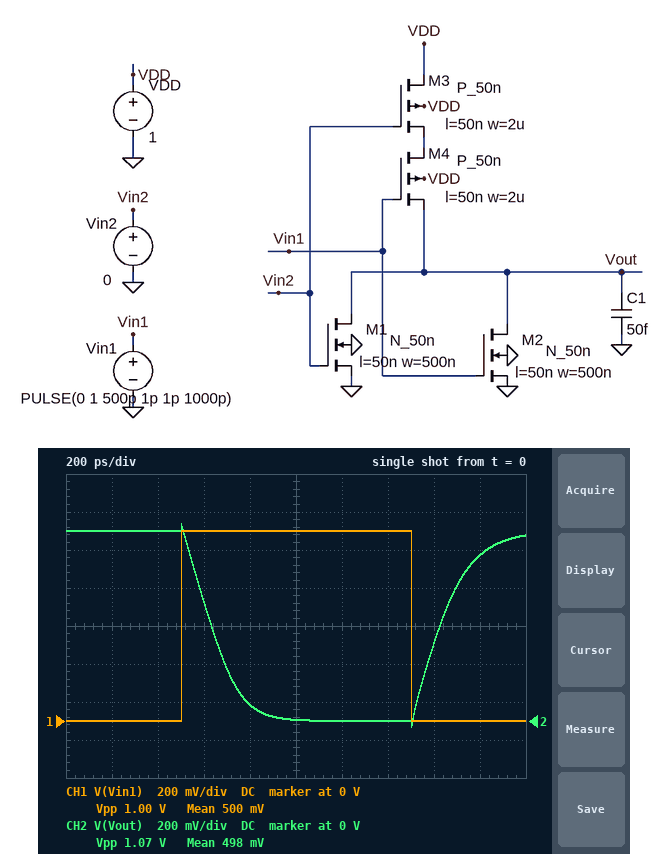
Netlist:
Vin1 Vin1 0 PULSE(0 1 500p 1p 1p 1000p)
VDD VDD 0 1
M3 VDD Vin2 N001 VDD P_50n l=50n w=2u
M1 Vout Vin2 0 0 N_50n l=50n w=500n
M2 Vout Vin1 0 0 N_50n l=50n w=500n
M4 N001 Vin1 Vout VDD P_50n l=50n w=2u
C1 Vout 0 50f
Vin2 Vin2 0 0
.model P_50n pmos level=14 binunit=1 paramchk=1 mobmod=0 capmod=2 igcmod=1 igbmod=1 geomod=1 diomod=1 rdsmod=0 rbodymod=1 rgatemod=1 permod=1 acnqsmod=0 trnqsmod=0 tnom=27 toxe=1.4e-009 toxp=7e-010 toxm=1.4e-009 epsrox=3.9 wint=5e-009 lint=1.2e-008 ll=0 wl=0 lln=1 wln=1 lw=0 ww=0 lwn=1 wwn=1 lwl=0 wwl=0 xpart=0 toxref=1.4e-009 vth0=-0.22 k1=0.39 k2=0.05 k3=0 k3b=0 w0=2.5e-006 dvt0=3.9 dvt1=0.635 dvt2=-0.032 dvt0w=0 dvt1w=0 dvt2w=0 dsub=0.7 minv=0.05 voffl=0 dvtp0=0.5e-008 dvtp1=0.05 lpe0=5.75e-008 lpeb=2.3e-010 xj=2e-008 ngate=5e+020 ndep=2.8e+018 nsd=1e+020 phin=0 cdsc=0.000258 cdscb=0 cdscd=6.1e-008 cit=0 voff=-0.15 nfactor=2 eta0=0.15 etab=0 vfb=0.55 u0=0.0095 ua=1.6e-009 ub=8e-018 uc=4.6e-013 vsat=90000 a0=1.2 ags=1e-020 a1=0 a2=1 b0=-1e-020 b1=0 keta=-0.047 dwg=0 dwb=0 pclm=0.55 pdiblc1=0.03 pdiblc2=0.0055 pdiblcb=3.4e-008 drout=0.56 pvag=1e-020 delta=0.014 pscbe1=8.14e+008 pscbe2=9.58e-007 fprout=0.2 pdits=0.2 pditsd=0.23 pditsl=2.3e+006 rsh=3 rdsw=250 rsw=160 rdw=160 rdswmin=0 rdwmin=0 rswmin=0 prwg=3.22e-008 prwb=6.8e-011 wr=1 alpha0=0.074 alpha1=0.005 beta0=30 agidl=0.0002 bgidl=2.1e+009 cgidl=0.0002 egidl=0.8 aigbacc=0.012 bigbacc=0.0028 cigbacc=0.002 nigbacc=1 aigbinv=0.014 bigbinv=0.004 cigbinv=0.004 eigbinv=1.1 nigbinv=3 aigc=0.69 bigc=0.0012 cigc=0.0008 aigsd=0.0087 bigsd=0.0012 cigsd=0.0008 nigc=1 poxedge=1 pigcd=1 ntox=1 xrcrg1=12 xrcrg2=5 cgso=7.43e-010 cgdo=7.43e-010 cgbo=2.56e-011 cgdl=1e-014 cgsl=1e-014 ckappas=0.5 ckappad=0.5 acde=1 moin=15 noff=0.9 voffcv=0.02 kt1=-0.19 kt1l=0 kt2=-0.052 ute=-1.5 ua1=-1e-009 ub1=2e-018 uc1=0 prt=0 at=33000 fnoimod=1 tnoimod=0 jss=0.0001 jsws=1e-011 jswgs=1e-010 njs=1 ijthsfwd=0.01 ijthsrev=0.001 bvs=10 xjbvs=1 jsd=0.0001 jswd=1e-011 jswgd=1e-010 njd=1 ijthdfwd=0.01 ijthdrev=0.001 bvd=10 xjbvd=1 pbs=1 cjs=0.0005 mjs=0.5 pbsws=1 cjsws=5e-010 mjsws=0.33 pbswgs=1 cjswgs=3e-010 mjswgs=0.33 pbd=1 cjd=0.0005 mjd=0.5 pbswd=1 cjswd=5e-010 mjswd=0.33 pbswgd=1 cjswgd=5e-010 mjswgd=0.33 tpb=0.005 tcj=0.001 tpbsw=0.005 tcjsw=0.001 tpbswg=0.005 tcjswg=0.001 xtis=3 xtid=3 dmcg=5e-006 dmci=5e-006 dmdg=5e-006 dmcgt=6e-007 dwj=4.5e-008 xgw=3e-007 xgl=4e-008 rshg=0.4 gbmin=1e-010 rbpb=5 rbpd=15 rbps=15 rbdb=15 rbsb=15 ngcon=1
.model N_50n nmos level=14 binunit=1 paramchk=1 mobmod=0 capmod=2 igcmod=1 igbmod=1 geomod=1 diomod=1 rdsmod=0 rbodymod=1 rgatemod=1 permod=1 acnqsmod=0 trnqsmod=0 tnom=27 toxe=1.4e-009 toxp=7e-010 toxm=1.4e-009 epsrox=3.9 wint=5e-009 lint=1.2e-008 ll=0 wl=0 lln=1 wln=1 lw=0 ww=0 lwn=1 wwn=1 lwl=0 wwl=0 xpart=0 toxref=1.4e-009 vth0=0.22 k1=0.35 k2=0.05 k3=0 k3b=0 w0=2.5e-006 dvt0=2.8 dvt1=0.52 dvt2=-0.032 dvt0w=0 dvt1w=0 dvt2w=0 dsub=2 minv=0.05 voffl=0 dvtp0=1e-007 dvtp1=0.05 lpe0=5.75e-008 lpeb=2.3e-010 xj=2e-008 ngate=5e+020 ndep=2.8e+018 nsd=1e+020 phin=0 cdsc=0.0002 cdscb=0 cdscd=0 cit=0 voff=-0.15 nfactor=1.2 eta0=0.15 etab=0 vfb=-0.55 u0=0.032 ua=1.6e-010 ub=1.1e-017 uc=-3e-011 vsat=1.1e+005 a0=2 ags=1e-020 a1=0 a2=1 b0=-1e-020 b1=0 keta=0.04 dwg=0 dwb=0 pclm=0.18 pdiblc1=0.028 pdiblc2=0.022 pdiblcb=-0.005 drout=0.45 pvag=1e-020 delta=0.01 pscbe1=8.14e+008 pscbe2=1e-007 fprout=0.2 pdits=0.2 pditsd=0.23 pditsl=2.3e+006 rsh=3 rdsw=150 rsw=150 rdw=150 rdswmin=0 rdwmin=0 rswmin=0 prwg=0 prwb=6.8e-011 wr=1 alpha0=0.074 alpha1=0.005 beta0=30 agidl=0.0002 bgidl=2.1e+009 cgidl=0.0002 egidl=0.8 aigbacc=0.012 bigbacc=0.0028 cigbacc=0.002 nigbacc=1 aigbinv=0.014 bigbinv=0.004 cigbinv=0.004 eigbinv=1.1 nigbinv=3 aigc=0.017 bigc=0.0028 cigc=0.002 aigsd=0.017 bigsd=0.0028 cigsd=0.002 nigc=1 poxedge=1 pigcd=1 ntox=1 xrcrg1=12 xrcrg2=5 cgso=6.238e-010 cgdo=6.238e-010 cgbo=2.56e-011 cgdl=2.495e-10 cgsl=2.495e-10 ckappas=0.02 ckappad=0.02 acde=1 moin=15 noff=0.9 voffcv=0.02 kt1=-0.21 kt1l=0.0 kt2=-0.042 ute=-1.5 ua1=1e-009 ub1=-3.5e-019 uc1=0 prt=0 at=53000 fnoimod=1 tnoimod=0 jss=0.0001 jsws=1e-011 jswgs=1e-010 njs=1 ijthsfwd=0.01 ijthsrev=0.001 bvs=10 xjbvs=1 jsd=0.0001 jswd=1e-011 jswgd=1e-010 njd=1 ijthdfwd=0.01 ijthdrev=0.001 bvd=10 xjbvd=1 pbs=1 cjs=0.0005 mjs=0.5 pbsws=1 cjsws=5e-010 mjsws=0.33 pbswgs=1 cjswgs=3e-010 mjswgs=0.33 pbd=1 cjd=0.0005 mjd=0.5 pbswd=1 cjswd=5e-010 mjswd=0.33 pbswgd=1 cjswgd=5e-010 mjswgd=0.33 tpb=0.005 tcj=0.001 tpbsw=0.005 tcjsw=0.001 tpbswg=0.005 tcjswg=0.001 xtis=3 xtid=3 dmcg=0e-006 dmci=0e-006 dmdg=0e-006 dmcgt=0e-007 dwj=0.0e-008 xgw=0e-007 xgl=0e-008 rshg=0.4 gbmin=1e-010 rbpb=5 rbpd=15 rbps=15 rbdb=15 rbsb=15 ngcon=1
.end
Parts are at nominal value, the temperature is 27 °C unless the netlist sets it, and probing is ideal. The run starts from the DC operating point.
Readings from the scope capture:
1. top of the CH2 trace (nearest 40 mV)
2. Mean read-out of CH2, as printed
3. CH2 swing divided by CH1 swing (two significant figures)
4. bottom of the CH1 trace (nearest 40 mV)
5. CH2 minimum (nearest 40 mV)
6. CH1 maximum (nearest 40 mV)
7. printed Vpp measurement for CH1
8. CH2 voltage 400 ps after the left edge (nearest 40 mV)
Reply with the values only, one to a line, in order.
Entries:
1.04 V
498 mV
1.1
0 V
-40 mV
1.00 V
1.00 V
1.00 V
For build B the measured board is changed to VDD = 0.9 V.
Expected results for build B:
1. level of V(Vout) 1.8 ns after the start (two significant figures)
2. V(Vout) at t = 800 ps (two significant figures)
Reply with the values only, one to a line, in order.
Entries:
760 mV
64 mV
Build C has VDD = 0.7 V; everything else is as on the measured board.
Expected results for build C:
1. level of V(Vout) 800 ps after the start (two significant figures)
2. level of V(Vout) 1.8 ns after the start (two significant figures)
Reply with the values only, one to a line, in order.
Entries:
35 mV
470 mV
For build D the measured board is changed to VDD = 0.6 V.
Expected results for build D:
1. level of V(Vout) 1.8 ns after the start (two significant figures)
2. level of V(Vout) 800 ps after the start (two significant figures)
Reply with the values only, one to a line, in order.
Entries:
290 mV
26 mV
